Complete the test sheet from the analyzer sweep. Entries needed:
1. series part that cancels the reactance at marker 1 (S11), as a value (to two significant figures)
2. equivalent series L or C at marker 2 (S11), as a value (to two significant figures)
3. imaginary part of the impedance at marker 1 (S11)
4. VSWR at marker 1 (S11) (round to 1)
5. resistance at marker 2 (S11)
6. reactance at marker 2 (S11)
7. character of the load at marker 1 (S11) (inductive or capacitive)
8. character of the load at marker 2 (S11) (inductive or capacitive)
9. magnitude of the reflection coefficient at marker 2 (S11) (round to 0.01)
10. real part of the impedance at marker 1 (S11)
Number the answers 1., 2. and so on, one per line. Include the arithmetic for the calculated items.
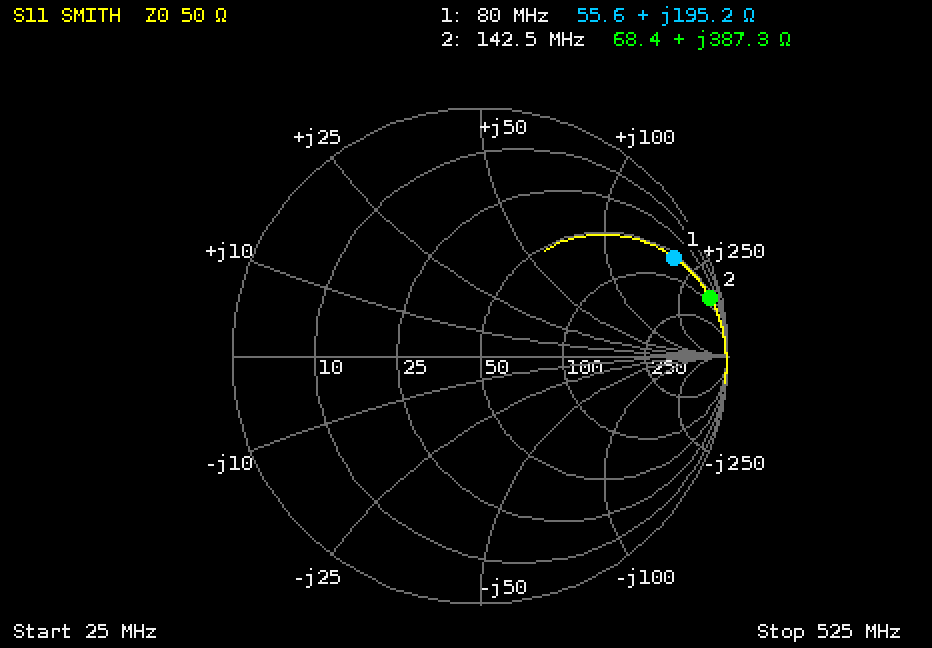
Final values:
1. C = 1/(2π × 80 MHz × 195.2 Ω) ≈ 10 pF
2. L = 387.3 Ω/(2π × 142.5 MHz) ≈ 433 nH, so 430 nH to two significant figures
3. +195.2 Ω
4. 16
5. 68.4 Ω
6. +387.3 Ω
7. inductive
8. inductive
9. 0.96
10. 55.6 Ω
